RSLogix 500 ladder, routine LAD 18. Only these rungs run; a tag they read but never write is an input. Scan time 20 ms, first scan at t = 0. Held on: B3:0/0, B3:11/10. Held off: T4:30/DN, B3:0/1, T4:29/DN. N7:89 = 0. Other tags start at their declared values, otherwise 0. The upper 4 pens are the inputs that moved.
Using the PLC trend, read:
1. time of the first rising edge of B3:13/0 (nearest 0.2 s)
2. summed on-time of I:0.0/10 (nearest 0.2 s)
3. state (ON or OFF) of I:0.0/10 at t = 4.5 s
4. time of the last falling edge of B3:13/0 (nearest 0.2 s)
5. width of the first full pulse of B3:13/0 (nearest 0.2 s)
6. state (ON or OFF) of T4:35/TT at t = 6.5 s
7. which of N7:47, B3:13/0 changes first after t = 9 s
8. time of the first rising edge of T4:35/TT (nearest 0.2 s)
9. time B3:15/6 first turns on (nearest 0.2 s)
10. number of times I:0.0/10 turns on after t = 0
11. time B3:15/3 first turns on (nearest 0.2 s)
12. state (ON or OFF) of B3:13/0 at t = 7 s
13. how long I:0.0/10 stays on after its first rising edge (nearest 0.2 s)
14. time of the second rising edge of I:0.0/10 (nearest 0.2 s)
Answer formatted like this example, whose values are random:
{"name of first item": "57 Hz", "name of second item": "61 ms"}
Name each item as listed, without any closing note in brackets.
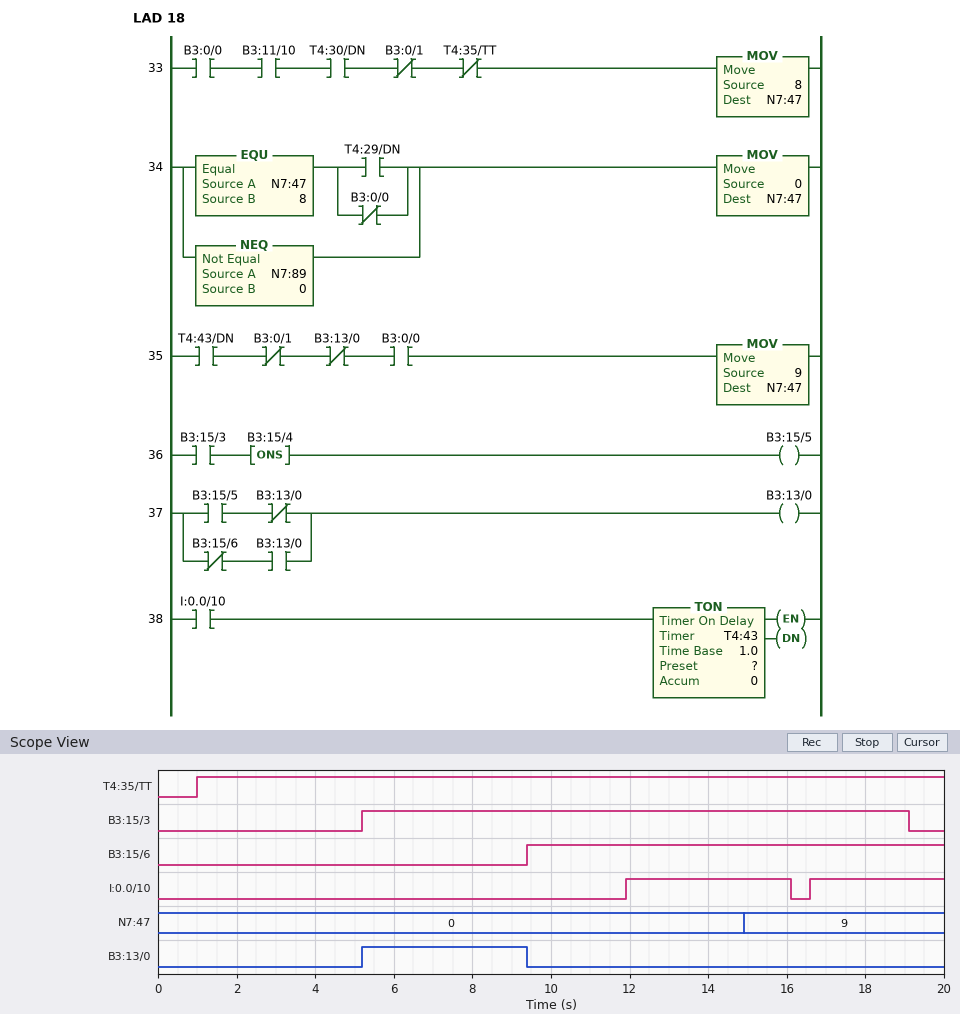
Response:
{"time of the first rising edge of B3:13/0": "5.2 s", "summed on-time of I:0.0/10": "7.6 s", "state (ON or OFF) of I:0.0/10 at t = 4.5 s": "OFF", "time of the last falling edge of B3:13/0": "9.4 s", "width of the first full pulse of B3:13/0": "4.2 s", "state (ON or OFF) of T4:35/TT at t = 6.5 s": "ON", "which of N7:47, B3:13/0 changes first after t = 9 s": "B3:13/0", "time of the first rising edge of T4:35/TT": "1.0 s", "time B3:15/6 first turns on": "9.4 s", "number of times I:0.0/10 turns on after t = 0": "2", "time B3:15/3 first turns on": "5.2 s", "state (ON or OFF) of B3:13/0 at t = 7 s": "ON", "how long I:0.0/10 stays on after its first rising edge": "4.2 s", "time of the second rising edge of I:0.0/10": "16.6 s"}
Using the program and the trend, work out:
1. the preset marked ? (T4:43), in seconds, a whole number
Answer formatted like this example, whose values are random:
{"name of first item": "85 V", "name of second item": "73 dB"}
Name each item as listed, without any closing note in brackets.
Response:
{"the preset marked ? (T4:43), in seconds, a whole number": "3 s"}
